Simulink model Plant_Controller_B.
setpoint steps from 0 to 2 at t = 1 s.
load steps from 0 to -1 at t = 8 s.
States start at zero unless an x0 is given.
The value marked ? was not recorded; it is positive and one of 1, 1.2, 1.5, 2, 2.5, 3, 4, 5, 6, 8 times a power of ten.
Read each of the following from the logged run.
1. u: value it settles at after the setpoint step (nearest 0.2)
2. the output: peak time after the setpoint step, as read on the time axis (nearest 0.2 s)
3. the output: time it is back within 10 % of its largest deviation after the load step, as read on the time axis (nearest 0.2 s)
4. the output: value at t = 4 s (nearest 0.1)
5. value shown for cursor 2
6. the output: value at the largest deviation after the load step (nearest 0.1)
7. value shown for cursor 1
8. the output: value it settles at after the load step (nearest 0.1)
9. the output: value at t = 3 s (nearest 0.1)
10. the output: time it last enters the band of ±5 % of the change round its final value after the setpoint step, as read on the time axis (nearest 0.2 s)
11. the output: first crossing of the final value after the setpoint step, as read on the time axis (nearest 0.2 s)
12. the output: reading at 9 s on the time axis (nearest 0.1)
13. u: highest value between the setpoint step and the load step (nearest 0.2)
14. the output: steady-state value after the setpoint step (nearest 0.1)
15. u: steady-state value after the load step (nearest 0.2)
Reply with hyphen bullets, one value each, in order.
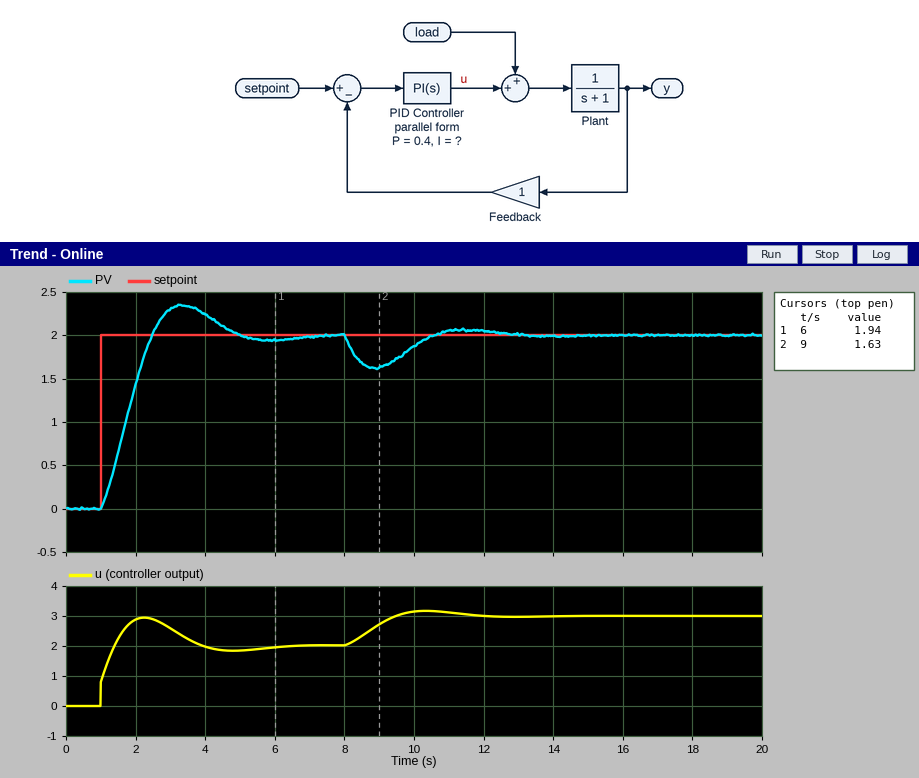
- 2.0
- 3.4 s
- 12.2 s
- 2.2
- 1.63
- 1.6
- 1.94
- 2.0
- 2.3
- 4.6 s
- 2.4 s
- 1.6
- 3.0
- 2.0
- 3.0
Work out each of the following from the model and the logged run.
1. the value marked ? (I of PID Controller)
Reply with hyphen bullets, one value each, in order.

- 2
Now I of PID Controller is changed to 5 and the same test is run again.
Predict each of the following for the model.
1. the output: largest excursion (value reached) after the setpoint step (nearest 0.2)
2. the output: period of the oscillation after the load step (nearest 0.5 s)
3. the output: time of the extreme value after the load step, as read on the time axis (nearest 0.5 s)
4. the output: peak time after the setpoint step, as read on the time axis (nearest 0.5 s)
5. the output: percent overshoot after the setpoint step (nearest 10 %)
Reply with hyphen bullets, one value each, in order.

- 2.8
- 3.0 s
- 8.5 s
- 2.5 s
- 40 %
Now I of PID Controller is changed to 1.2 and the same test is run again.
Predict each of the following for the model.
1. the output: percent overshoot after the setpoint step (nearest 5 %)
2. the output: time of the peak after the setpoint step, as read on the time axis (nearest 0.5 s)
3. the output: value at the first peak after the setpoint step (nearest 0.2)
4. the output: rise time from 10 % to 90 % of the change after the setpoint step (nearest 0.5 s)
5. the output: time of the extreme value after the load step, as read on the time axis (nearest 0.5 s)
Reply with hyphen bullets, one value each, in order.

- 10 %
- 4.5 s
- 2.2
- 1.5 s
- 9.0 s
